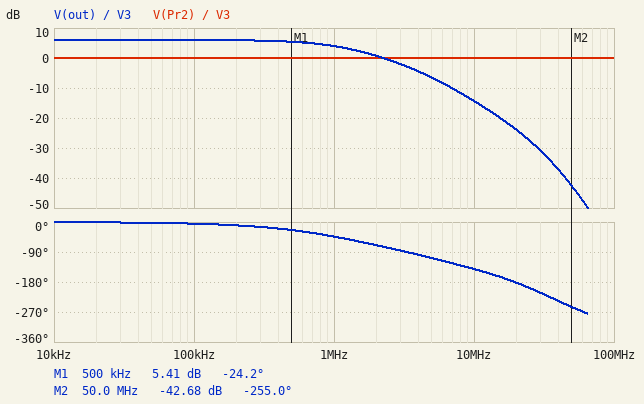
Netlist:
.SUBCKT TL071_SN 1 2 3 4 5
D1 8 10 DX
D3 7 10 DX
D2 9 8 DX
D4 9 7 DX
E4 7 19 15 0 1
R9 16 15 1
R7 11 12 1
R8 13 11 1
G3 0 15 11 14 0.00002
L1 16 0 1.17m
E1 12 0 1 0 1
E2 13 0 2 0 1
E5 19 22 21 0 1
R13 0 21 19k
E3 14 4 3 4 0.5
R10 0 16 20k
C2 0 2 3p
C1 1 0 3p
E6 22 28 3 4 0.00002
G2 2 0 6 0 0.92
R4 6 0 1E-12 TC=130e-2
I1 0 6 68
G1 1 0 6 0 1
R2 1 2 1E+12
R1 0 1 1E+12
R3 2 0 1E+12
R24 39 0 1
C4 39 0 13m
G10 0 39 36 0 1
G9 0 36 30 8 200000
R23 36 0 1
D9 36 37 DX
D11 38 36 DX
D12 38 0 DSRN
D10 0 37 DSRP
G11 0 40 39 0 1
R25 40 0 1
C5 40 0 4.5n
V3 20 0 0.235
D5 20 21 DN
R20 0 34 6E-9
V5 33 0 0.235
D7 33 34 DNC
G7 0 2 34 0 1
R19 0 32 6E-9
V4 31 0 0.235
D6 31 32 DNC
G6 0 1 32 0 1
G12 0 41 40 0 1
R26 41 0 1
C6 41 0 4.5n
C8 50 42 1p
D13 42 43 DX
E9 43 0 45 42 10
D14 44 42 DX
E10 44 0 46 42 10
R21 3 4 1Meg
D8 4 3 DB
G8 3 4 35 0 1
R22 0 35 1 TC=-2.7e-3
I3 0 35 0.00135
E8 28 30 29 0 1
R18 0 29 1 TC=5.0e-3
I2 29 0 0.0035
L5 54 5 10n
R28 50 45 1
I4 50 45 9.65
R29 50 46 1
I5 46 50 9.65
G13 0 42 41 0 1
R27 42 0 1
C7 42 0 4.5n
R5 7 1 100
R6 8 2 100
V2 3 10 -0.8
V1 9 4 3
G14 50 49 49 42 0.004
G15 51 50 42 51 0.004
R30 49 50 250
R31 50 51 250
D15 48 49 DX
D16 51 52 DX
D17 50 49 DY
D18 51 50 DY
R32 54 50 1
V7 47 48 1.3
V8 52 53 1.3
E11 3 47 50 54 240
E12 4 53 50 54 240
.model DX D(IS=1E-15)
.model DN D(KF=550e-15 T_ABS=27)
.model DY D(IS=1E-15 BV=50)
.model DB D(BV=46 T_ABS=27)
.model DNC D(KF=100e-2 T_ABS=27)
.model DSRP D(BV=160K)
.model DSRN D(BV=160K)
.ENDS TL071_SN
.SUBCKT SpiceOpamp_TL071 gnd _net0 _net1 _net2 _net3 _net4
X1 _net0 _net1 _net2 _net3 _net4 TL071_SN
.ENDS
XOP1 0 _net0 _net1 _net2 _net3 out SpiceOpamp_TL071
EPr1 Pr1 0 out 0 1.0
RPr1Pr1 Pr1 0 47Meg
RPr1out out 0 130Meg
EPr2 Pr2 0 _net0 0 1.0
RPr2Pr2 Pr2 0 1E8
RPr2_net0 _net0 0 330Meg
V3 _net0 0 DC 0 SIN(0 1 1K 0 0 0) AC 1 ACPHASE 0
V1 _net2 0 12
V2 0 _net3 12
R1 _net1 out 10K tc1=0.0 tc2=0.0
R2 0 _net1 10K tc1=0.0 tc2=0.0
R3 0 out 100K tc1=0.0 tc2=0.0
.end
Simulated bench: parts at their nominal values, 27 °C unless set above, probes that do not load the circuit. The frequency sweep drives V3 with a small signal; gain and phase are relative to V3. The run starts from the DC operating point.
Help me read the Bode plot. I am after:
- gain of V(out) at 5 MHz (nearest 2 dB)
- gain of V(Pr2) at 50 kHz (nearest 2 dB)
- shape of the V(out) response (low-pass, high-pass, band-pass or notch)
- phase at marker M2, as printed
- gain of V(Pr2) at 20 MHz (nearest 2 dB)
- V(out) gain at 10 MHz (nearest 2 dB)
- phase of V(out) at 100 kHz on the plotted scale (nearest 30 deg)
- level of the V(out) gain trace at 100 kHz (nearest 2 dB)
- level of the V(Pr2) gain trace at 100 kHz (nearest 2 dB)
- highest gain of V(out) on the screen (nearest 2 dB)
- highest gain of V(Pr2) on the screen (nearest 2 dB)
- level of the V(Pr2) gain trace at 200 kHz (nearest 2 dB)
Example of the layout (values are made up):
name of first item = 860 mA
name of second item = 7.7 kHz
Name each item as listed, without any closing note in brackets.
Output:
gain of V(out) at 5 MHz = -6 dB
gain of V(Pr2) at 50 kHz = 0 dB
shape of the V(out) response = low-pass
phase at marker M2, as printed = -255.0 deg
gain of V(Pr2) at 20 MHz = 0 dB
V(out) gain at 10 MHz = -14 dB
phase of V(out) at 100 kHz on the plotted scale = 0 deg
level of the V(out) gain trace at 100 kHz = 6 dB
level of the V(Pr2) gain trace at 100 kHz = 0 dB
highest gain of V(out) on the screen = 6 dB
highest gain of V(Pr2) on the screen = 0 dB
level of the V(Pr2) gain trace at 200 kHz = 0 dB
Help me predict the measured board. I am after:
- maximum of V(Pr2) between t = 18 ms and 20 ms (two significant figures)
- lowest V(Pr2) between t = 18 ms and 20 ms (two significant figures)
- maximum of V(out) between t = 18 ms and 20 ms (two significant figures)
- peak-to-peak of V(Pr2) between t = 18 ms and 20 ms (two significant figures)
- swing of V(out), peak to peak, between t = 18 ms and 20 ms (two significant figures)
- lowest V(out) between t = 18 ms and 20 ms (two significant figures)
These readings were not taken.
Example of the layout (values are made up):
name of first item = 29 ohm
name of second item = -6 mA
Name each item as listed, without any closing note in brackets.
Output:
maximum of V(Pr2) between t = 18 ms and 20 ms = 1.0 V
lowest V(Pr2) between t = 18 ms and 20 ms = -1.0 V
maximum of V(out) between t = 18 ms and 20 ms = 2.0 V
peak-to-peak of V(Pr2) between t = 18 ms and 20 ms = 2.0 V
swing of V(out), peak to peak, between t = 18 ms and 20 ms = 4.0 V
lowest V(out) between t = 18 ms and 20 ms = -2.0 V
